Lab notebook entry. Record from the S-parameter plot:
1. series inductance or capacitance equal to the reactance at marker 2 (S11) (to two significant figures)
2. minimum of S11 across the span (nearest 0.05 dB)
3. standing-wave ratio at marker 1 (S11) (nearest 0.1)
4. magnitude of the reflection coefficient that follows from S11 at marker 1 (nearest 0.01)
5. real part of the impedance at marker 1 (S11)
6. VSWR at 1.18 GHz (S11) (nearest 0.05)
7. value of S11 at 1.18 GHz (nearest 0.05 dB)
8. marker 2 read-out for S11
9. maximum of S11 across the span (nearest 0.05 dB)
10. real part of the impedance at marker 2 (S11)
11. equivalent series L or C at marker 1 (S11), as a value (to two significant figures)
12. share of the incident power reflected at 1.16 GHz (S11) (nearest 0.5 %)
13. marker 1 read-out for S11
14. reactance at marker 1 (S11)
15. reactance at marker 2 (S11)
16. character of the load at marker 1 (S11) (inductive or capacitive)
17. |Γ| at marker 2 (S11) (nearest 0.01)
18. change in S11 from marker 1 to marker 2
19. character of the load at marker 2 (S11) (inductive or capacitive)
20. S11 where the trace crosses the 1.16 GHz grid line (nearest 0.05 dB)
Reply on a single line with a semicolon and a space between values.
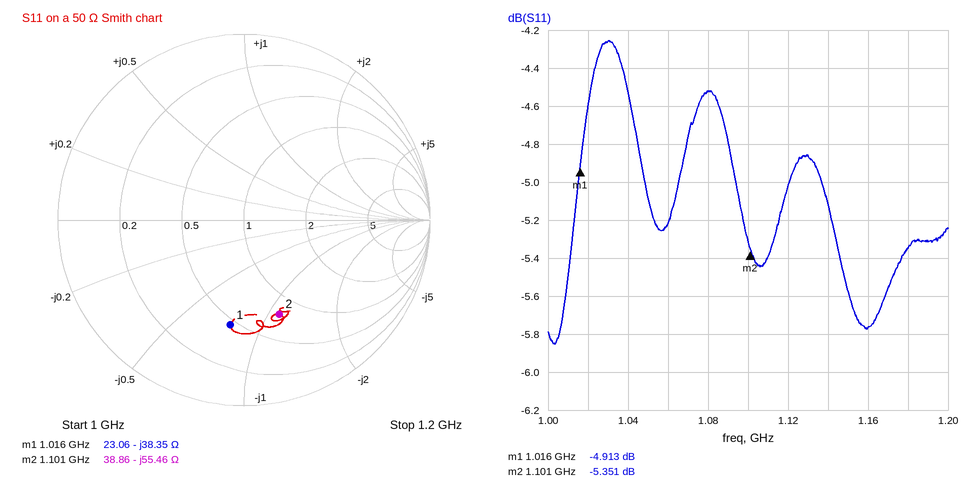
2.6 pF; -5.85 dB; 3.6; 0.57; 23.06 Ω; 3.35; -5.35 dB; -5.351 dB; -4.25 dB; 38.86 Ω; 4.1 pF; 26.5 %; -4.913 dB; -38.35 Ω; -55.46 Ω; capacitive; 0.54; -0.438 dB; capacitive; -5.75 dB
